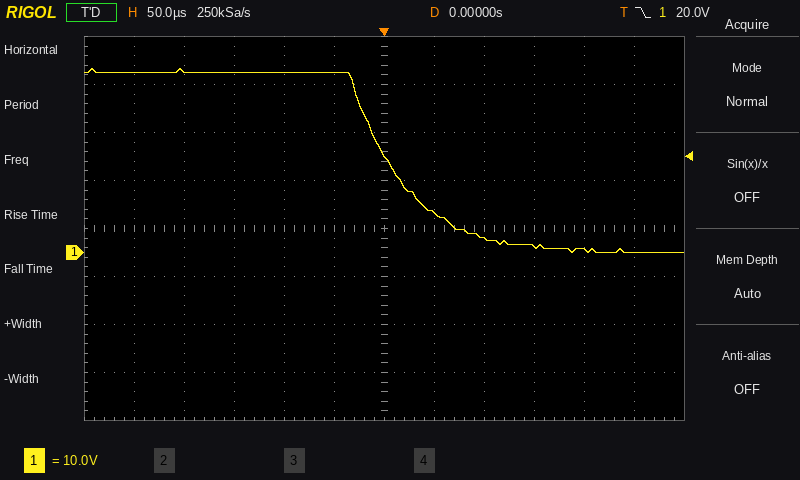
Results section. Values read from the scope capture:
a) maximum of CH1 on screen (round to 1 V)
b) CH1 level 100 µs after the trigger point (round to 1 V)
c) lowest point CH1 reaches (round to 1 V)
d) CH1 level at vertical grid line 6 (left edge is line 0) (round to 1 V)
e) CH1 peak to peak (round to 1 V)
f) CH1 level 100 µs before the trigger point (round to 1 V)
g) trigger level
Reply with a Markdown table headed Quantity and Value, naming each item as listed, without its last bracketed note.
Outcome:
| Quantity | Value |
|---|---|
| maximum of CH1 on screen | 38 V |
| CH1 level 100 µs after the trigger point | 3 V |
| lowest point CH1 reaches | 0 V |
| CH1 level at vertical grid line 6 (left edge is line 0) | 20 V |
| CH1 peak to peak | 38 V |
| CH1 level 100 µs before the trigger point | 38 V |
| trigger level | 20.0 V |
